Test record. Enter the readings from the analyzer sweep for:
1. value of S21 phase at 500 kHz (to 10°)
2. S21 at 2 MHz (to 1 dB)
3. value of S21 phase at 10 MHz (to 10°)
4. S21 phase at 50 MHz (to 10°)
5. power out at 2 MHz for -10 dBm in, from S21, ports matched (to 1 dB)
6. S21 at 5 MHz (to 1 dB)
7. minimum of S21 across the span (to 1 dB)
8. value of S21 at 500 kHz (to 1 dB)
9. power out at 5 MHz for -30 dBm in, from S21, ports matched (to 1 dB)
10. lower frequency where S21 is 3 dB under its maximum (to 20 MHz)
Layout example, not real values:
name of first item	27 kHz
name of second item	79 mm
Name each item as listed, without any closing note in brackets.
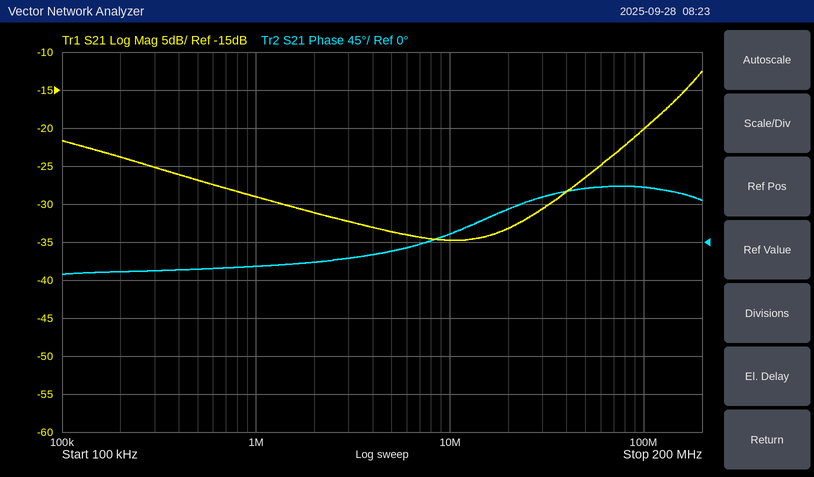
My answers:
value of S21 phase at 500 kHz	-30°
S21 at 2 MHz	-31 dB
value of S21 phase at 10 MHz	10°
S21 phase at 50 MHz	60°
power out at 2 MHz for -10 dBm in, from S21, ports matched	-41 dBm
S21 at 5 MHz	-34 dB
minimum of S21 across the span	-35 dB
value of S21 at 500 kHz	-27 dB
power out at 5 MHz for -30 dBm in, from S21, ports matched	-64 dBm
lower frequency where S21 is 3 dB under its maximum	160 MHz
